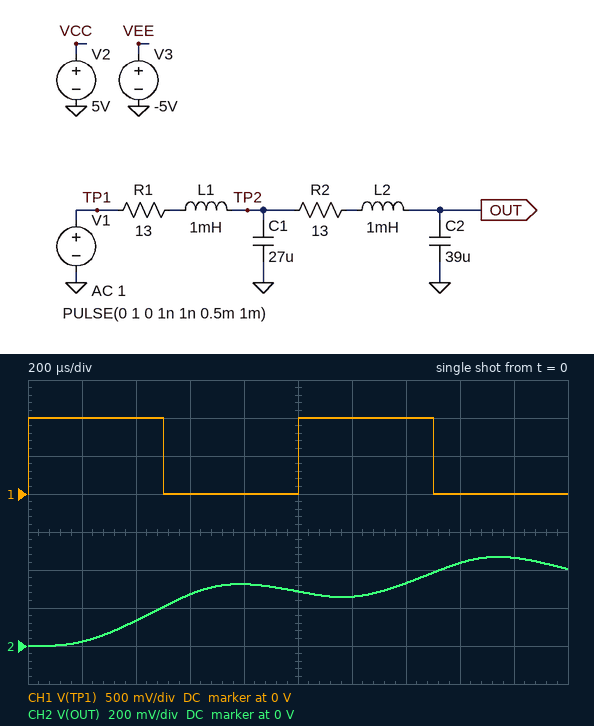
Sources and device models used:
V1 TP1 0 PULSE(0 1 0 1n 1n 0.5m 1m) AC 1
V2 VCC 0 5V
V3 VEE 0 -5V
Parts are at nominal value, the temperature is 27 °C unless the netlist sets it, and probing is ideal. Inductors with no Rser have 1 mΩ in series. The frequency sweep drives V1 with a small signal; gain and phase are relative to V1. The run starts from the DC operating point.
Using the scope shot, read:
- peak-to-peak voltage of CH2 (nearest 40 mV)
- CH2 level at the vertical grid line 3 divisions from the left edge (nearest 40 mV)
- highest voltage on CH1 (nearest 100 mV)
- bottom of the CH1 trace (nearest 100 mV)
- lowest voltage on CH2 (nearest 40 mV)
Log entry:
480 mV
280 mV
1.0 V
0 V
0 V
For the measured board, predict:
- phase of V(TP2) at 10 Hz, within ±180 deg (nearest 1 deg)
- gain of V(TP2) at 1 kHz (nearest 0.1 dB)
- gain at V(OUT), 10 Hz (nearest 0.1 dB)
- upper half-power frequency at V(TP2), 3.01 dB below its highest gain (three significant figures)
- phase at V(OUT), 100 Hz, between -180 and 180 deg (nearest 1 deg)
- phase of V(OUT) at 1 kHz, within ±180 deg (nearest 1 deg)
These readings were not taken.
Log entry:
-3 deg
-8.6 dB
0 dB
164 Hz
-44 deg
-168 deg
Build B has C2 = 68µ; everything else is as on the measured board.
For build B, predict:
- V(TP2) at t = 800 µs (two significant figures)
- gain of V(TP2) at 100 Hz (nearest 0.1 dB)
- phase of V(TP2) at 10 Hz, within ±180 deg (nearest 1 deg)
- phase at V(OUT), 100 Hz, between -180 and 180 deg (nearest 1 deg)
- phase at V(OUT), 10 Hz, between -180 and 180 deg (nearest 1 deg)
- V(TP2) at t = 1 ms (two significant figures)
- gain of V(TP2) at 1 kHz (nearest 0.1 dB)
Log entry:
160 mV
-2.8 dB
-4 deg
-58 deg
-8 deg
95 mV
-8.2 dB
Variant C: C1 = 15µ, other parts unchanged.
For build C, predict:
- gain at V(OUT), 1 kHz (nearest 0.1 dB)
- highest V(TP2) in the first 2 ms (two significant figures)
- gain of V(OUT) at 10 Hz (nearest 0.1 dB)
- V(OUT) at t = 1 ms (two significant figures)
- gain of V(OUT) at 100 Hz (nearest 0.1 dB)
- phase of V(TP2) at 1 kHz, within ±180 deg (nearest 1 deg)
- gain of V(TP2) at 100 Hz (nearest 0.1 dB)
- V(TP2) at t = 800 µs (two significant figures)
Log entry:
-16.7 dB
700 mV
0 dB
280 mV
-1.5 dB
-46 deg
-1.2 dB
130 mV
